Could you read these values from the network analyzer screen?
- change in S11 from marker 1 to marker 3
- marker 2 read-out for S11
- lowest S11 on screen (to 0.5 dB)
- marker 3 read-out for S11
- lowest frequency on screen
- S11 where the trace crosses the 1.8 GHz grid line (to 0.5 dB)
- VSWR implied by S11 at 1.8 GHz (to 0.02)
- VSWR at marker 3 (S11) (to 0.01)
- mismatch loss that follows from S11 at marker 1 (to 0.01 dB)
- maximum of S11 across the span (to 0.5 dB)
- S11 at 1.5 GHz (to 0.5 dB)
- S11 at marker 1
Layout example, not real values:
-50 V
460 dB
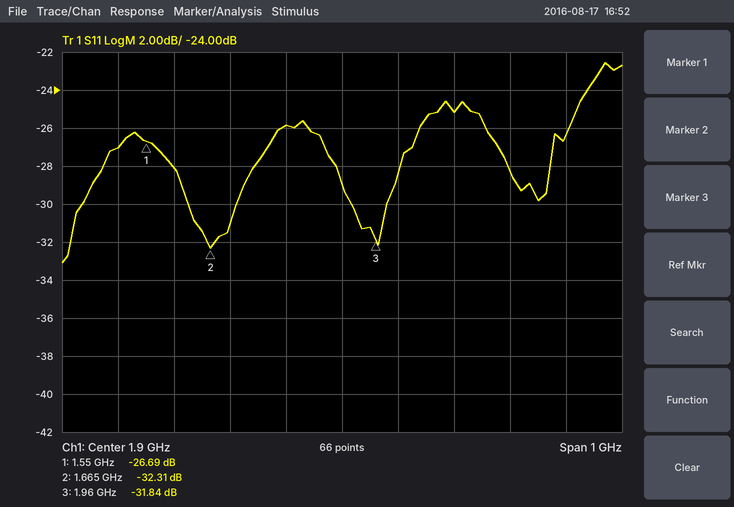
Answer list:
-5.15 dB
-32.31 dB
-33.0 dB
-31.84 dB
1.4 GHz
-26.0 dB
1.10
1.05
0.01 dB
-22.5 dB
-27.0 dB
-26.69 dB
